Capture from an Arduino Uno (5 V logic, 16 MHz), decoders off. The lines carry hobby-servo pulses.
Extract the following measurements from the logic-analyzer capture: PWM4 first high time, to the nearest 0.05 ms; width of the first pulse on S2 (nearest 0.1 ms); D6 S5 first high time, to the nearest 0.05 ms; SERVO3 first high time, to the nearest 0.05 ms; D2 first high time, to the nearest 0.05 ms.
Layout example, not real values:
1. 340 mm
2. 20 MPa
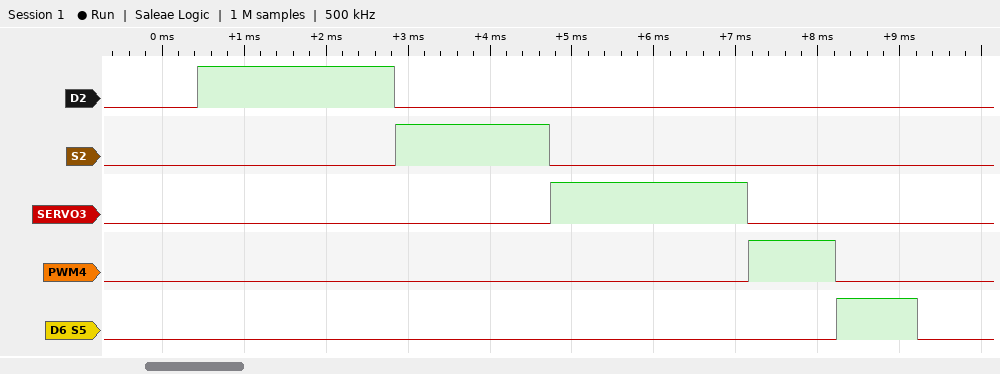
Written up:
1. 1.05 ms
2. 1.9 ms
3. 1.00 ms
4. 2.40 ms
5. 2.40 ms
